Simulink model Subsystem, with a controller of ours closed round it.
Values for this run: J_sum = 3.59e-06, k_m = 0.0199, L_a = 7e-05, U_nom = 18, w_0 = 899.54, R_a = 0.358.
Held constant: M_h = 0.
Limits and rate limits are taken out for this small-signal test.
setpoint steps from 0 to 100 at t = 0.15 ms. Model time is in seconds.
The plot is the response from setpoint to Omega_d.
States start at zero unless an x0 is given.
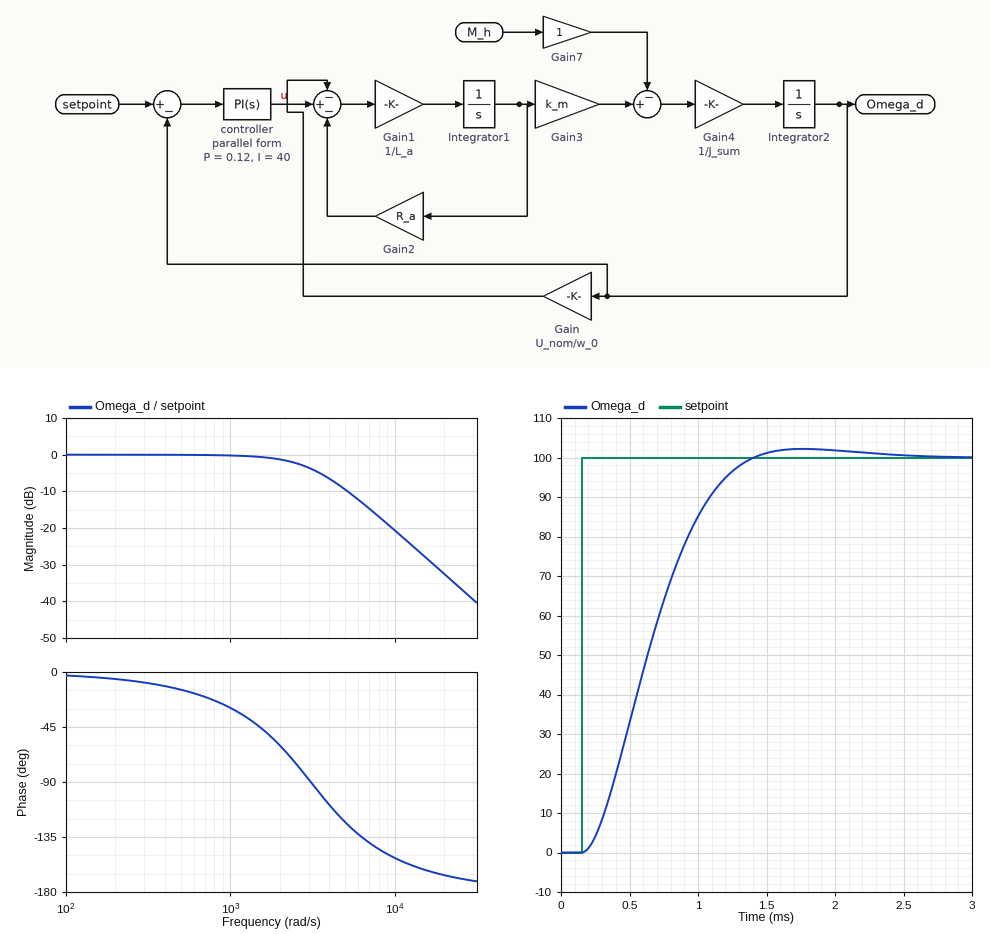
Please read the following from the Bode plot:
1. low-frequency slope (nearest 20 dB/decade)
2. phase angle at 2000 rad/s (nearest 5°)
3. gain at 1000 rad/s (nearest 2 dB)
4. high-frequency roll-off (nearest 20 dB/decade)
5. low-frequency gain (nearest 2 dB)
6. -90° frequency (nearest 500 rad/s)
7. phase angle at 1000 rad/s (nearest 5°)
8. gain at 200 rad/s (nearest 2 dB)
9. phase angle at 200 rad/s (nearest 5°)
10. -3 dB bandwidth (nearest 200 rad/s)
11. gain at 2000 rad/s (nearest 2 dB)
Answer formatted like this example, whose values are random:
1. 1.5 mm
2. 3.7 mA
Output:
1. 0 dB/decade
2. -60°
3. 0 dB
4. -40 dB/decade
5. 0 dB
6. 3000 rad/s
7. -30°
8. 0 dB
9. -5°
10. 2800 rad/s
11. -2 dB
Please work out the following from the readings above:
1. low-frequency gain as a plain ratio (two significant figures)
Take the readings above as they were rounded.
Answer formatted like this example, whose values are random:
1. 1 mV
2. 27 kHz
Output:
1. 1.0
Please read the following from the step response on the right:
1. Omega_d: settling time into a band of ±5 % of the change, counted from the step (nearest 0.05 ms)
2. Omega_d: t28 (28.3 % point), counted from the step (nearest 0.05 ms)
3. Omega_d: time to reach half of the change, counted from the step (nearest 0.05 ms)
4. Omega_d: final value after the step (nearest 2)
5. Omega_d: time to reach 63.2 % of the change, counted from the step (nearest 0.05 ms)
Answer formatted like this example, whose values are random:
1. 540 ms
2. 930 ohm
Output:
1. 1.05 ms
2. 0.30 ms
3. 0.50 ms
4. 100
5. 0.60 ms
